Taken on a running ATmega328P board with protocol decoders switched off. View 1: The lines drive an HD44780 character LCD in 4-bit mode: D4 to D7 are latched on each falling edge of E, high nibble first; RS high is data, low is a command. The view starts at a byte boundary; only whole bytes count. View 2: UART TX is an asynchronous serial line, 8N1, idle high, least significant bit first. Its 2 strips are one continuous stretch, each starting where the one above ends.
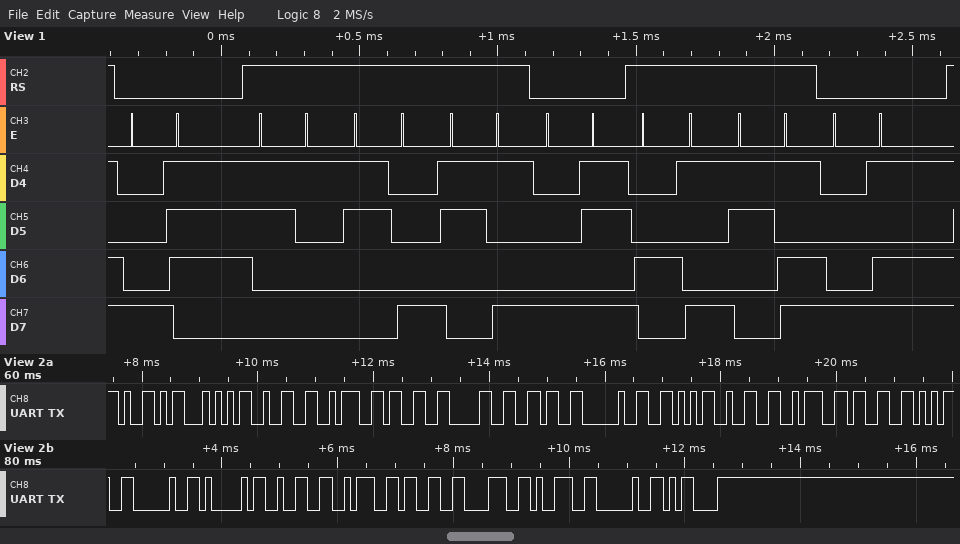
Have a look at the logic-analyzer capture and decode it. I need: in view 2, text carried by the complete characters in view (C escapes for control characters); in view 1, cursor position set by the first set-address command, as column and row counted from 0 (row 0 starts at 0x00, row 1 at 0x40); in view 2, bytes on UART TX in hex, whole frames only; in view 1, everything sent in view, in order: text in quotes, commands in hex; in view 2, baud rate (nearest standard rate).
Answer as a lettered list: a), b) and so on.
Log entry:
a) "YT2:306 V2:35 A2:389 \r"
b) column 7, row 0
c) 59 54 32 3A 33 30 36 20 56 32 3A 33 35 20 41 32 3A 33 38 39 20 0D
d) 0x87 "189" 0x8B "I=" 0x8D
e) 9600 baud
